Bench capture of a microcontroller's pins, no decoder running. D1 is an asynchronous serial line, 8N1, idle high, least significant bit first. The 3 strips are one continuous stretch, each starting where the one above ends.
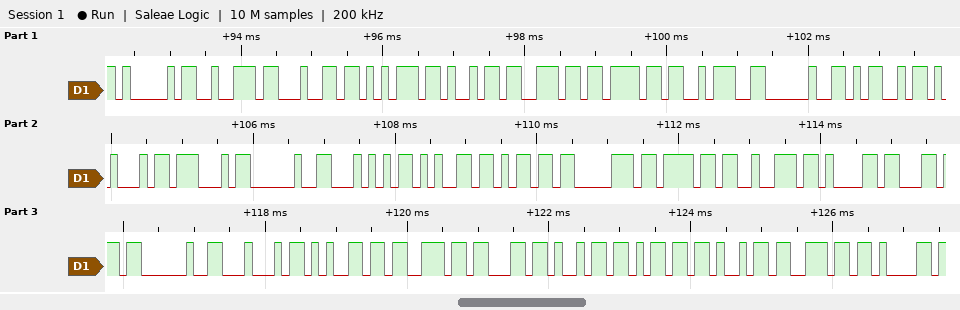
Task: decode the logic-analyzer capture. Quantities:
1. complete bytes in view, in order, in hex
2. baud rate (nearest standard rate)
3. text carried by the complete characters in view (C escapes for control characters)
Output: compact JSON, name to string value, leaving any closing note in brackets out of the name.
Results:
{"complete bytes in view, in order, in hex": "0x41 0x72 0x64 0x75 0x69 0x6E 0x6F 0x3A 0x20 0x4D 0x45 0x47 0x20 0x54 0x65 0x6D 0x70 0x6F 0x72 0x61 0x6C 0x20 0x44 0x65 0x73 0x63 0x69 0x6D 0x69 0x6E 0x61", "baud rate": "9600 baud", "text carried by the complete characters in view": "\"Arduino: MEG Temporal Descimina\""}
